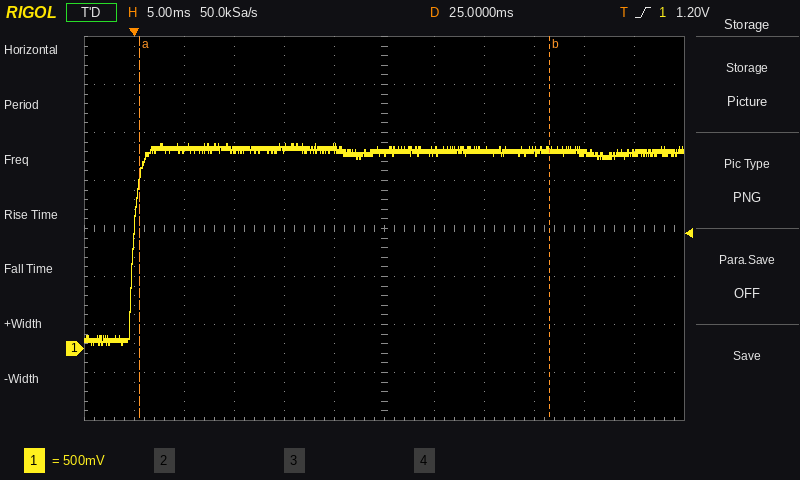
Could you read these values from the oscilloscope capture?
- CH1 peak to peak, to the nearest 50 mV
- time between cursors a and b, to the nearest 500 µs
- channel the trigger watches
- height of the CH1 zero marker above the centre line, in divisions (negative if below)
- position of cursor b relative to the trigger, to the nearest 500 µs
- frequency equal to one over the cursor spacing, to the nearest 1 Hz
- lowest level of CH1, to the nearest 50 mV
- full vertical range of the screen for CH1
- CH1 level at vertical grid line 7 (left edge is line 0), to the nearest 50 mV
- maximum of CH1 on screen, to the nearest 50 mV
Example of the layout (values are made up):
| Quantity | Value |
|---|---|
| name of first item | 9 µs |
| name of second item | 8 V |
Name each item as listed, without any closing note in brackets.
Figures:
| Quantity | Value |
|---|---|
| CH1 peak to peak, to the nearest 50 mV | 2.10 V |
| time between cursors a and b, to the nearest 500 µs | 41.0 ms |
| channel the trigger watches | CH1 |
| height of the CH1 zero marker above the centre line, in divisions | -2.5 div |
| position of cursor b relative to the trigger, to the nearest 500 µs | +41.5 ms |
| frequency equal to one over the cursor spacing, to the nearest 1 Hz | 24 Hz |
| lowest level of CH1, to the nearest 50 mV | 50 mV |
| full vertical range of the screen for CH1 | 4 V |
| CH1 level at vertical grid line 7 (left edge is line 0), to the nearest 50 mV | 2.05 V |
| maximum of CH1 on screen, to the nearest 50 mV | 2.15 V |
